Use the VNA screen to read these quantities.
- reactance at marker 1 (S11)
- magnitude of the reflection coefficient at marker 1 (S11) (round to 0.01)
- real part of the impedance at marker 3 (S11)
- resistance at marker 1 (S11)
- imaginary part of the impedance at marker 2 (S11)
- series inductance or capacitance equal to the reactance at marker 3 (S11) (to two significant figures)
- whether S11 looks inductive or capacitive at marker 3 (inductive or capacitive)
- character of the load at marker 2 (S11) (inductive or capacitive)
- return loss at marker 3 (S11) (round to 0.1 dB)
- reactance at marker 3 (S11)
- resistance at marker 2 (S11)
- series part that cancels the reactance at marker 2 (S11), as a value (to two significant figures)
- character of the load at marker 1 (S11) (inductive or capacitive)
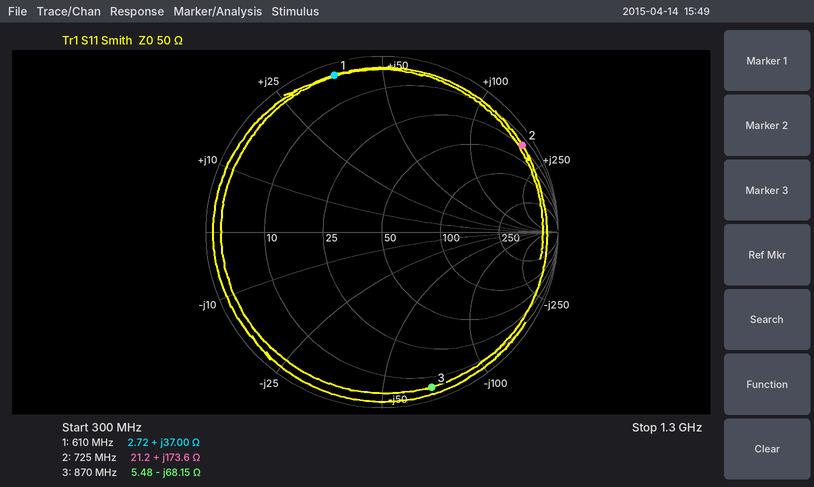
+37.00 Ω
0.93
5.48 Ω
2.72 Ω
+173.6 Ω
2.7 pF
capacitive
inductive
0.7 dB
-68.15 Ω
21.2 Ω
1.3 pF
inductive
